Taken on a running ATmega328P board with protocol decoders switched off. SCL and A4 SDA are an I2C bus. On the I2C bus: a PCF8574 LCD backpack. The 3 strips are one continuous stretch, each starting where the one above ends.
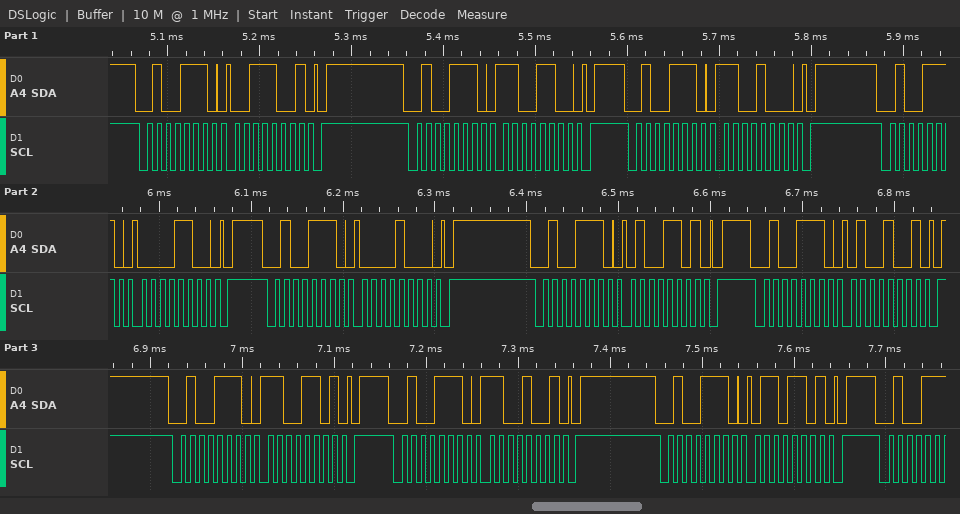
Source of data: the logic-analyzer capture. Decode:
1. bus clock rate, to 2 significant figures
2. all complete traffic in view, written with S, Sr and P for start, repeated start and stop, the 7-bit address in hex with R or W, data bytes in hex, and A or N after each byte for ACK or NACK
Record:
100 kHz
S 27W A 39 A P S 27W A CC A P S 27W A C8 A P S 27W A 0C A P S 27W A 08 A P S 27W A 4D A P S 27W A 49 A P S 27W A CD A P S 27W A C9 A P S 27W A 6D A P
